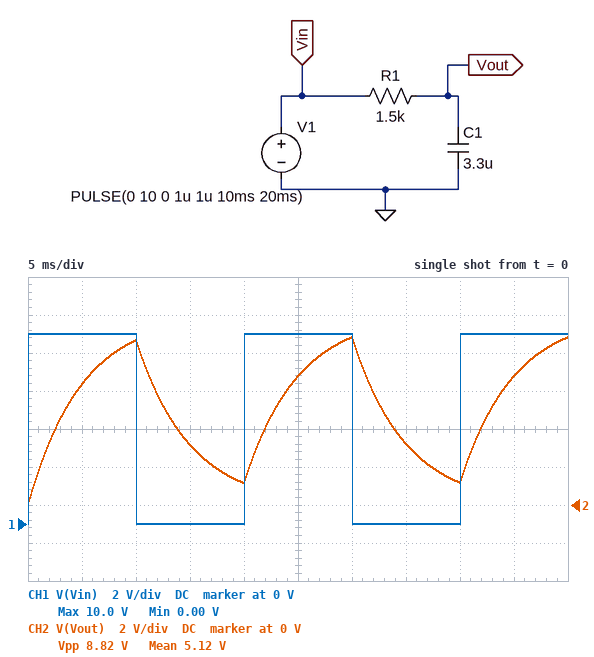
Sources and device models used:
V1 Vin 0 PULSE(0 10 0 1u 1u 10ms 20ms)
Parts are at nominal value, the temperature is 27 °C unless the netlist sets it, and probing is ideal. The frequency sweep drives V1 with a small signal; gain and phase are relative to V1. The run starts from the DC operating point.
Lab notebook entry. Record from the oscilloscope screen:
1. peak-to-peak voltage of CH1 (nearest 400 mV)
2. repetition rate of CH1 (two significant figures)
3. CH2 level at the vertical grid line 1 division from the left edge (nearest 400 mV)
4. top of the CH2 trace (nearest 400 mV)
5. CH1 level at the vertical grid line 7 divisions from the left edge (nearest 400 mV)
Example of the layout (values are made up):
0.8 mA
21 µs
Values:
10.0 V
50 Hz
6.4 V
8.8 V
0 V
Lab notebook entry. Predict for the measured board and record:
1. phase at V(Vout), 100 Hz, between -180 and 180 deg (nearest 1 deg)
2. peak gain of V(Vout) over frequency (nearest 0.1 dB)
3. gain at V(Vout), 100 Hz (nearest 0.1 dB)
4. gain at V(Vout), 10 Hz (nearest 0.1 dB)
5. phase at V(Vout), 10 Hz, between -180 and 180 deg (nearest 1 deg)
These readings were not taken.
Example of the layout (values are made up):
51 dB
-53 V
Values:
-72 deg
0 dB
-10.3 dB
-0.4 dB
-17 deg
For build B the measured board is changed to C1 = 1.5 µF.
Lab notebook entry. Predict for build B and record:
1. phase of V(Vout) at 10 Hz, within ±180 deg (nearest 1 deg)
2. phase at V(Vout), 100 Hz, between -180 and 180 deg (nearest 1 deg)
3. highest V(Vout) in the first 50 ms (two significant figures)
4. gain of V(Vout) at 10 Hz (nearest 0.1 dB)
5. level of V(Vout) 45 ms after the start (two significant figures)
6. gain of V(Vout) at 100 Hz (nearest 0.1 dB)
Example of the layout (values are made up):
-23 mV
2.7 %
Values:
-8 deg
-55 deg
9.9 V
-0.1 dB
8.9 V
-4.8 dB
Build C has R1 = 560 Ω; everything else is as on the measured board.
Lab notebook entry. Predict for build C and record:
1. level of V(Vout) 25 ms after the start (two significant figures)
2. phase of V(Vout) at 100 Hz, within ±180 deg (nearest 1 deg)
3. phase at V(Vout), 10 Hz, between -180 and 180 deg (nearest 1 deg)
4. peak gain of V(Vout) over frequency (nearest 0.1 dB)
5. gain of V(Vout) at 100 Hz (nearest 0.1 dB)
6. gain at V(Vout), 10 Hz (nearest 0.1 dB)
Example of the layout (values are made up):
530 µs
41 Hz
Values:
9.3 V
-49 deg
-7 deg
0 dB
-3.7 dB
-0.1 dB
